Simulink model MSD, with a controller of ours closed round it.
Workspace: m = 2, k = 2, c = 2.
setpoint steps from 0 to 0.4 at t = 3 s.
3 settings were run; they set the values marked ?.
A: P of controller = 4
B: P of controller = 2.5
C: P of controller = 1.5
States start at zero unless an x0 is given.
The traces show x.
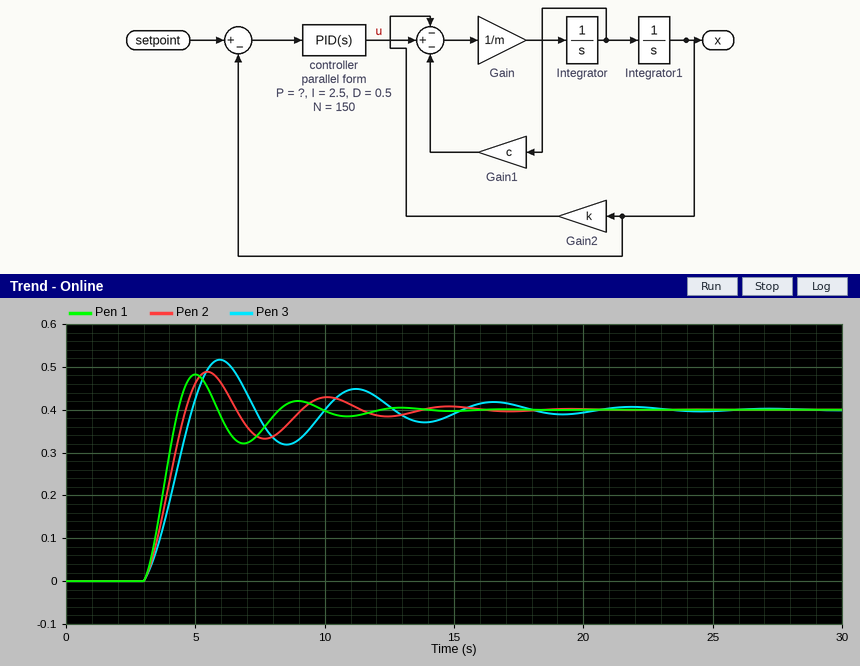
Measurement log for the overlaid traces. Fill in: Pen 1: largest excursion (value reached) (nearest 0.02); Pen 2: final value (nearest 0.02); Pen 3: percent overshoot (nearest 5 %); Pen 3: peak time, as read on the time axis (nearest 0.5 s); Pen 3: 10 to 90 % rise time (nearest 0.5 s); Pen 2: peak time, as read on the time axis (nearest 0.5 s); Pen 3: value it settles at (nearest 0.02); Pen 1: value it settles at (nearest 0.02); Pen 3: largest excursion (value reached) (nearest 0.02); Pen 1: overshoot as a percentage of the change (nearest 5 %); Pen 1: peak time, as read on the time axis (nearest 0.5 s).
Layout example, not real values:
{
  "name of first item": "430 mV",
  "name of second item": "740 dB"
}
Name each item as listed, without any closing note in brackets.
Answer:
{
  "Pen 1: largest excursion (value reached)": "0.48",
  "Pen 2: final value": "0.40",
  "Pen 3: percent overshoot": "30 %",
  "Pen 3: peak time, as read on the time axis": "6.0 s",
  "Pen 3: 10 to 90 % rise time": "1.5 s",
  "Pen 2: peak time, as read on the time axis": "5.5 s",
  "Pen 3: value it settles at": "0.40",
  "Pen 1: value it settles at": "0.40",
  "Pen 3: largest excursion (value reached)": "0.52",
  "Pen 1: overshoot as a percentage of the change": "20 %",
  "Pen 1: peak time, as read on the time axis": "5.0 s"
}
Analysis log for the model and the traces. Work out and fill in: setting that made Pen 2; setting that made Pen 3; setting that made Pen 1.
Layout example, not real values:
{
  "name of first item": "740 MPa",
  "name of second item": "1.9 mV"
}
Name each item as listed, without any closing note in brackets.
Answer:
{
  "setting that made Pen 2": "B",
  "setting that made Pen 3": "C",
  "setting that made Pen 1": "A"
}
